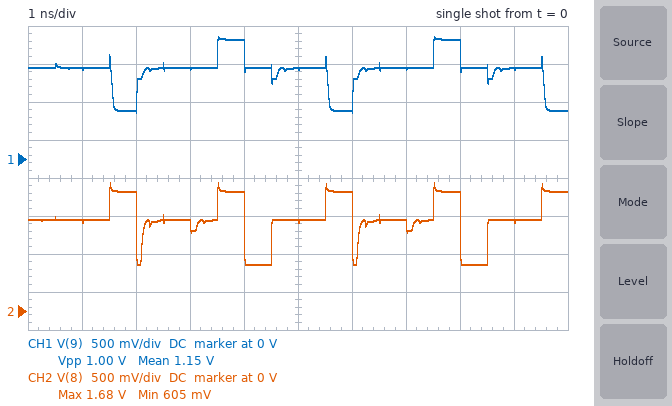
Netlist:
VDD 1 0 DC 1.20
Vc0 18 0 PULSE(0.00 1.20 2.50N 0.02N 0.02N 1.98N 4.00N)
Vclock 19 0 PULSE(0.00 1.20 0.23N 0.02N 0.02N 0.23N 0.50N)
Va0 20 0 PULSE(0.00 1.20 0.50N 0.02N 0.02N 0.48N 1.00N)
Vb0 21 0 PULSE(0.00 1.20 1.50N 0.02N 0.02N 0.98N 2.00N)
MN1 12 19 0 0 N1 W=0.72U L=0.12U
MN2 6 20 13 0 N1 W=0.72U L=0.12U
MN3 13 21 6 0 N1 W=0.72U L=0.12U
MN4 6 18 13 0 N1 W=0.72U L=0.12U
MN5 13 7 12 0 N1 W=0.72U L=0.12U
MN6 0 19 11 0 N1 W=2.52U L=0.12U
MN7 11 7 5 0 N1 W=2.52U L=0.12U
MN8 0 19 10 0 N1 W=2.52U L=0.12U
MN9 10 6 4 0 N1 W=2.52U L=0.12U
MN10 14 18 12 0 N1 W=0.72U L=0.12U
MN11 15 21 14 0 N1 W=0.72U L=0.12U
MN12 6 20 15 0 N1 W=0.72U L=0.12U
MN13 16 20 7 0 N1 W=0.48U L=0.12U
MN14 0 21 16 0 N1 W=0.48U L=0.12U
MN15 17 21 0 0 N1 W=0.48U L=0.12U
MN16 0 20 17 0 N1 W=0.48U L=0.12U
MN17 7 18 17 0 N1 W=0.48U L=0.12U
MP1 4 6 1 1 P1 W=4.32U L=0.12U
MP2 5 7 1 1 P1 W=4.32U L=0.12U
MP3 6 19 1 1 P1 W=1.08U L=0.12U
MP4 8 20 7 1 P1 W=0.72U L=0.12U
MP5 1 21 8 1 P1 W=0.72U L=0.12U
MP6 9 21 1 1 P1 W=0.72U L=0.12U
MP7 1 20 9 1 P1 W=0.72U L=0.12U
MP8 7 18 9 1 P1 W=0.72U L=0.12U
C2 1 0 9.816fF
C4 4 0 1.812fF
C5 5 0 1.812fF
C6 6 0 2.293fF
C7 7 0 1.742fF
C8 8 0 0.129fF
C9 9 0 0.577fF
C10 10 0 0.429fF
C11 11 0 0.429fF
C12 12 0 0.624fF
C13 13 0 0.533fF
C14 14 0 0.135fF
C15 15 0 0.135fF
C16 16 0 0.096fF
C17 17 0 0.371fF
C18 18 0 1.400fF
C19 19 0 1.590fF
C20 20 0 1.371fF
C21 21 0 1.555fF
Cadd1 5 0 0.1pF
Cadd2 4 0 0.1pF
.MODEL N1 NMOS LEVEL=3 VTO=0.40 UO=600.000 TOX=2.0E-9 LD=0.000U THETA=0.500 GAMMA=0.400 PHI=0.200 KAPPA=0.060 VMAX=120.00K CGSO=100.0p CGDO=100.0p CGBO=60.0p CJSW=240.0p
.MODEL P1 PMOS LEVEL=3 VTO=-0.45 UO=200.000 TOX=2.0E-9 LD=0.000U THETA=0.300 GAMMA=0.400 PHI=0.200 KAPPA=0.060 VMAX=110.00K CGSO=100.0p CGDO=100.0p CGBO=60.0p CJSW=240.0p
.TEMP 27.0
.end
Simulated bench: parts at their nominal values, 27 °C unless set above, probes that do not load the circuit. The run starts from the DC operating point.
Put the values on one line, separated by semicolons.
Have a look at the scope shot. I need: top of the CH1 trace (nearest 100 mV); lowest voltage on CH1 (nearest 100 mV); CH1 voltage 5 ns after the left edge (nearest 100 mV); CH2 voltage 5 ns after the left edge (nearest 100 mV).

1.6 V; 600 mV; 1.2 V; 1.2 V
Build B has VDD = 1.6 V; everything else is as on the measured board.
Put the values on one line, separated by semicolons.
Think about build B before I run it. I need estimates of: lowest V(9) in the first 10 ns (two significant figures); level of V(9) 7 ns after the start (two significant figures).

690 mV; 1.6 V
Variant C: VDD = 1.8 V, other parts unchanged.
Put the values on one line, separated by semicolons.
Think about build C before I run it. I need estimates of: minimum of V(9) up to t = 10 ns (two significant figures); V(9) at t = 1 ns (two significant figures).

900 mV; 1.8 V
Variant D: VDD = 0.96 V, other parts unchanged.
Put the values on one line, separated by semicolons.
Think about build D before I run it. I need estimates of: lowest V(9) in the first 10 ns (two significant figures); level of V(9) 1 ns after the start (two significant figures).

550 mV; 960 mV
